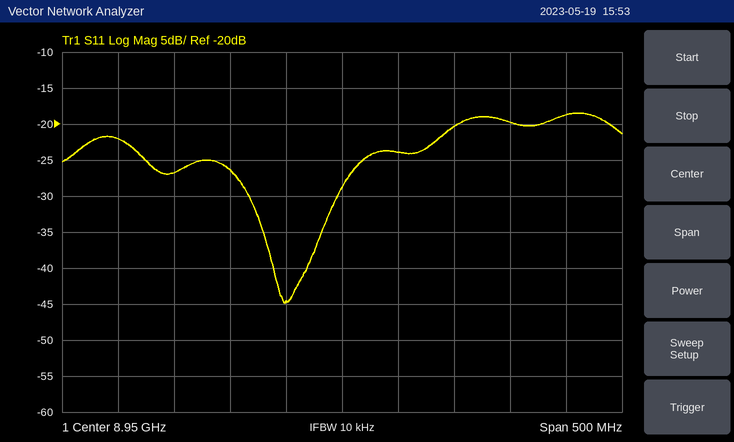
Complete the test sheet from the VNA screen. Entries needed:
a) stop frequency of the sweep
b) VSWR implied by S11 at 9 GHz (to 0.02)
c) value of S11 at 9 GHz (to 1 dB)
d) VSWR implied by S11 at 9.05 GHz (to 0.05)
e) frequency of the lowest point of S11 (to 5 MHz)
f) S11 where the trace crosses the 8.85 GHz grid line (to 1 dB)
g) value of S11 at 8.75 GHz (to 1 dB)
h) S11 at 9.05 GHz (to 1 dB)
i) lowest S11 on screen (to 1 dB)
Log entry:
9.2 GHz
1.14
-24 dB
1.20
8.900 GHz
-26 dB
-22 dB
-20 dB
-45 dB
